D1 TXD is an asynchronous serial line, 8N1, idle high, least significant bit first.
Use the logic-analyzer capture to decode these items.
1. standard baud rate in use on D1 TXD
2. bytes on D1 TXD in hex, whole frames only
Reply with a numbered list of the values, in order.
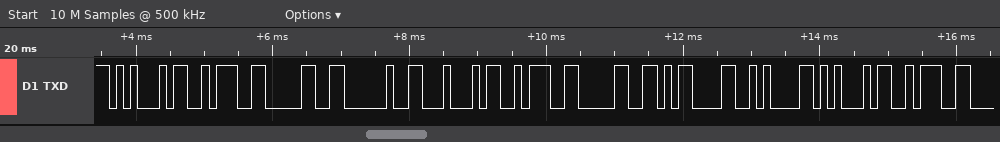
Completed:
1. 9600 baud
2. 0x45 0x3A 0x30 0x20 0x44 0x3A 0x30 0x0D 0x0A 0x45 0x3A
